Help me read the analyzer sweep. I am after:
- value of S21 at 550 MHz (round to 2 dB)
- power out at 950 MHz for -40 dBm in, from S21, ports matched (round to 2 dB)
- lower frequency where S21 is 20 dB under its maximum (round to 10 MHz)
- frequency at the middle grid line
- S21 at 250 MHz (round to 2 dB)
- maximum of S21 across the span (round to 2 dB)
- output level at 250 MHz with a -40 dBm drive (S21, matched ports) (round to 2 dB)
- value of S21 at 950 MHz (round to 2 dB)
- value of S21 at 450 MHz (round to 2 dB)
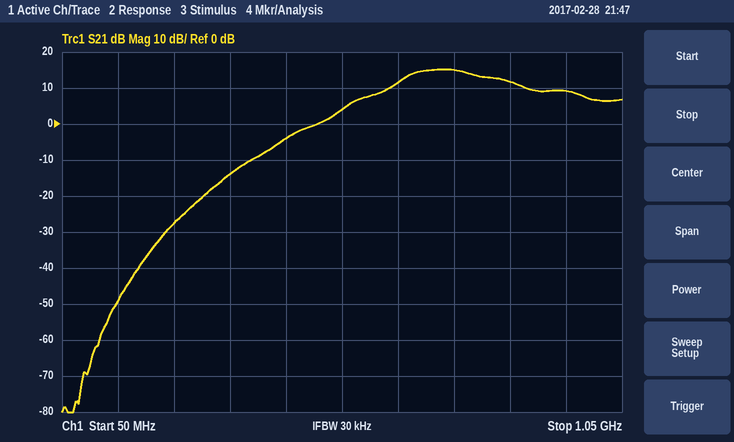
4 dB
-30 dBm
440 MHz
550 MHz
-28 dB
16 dB
-68 dBm
10 dB
-4 dB
